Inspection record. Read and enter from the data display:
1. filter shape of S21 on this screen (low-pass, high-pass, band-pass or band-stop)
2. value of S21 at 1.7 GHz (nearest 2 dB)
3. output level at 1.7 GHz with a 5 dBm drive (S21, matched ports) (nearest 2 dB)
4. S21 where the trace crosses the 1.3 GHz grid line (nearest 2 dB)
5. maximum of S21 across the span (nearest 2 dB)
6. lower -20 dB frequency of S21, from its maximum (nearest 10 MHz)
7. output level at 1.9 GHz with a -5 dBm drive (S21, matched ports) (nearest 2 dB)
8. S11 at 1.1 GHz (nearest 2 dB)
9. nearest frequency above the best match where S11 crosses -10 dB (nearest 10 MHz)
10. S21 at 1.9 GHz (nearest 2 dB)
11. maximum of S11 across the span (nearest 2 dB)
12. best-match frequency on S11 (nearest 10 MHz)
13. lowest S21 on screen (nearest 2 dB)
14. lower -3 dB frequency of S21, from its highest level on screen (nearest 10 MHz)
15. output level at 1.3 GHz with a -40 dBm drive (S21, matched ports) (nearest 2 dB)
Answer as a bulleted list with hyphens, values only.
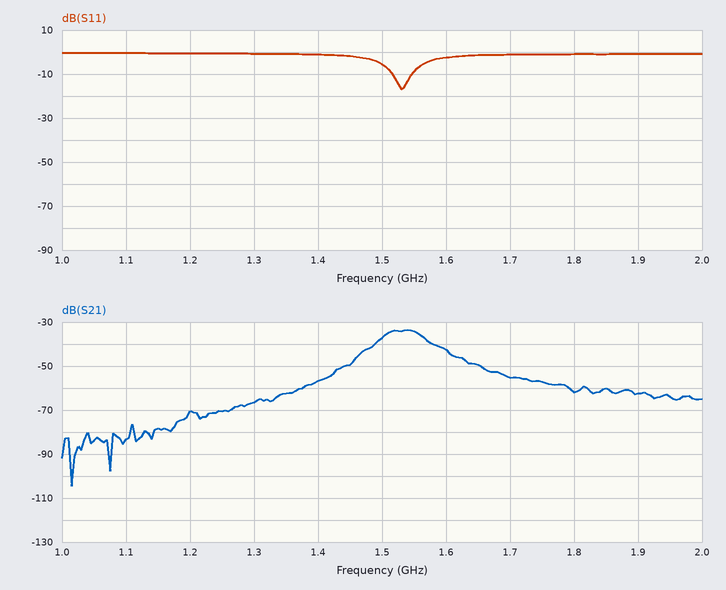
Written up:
- band-pass
- -56 dB
- -50 dBm
- -66 dB
- -34 dB
- 1.42 GHz
- -68 dBm
- 0 dB
- 1.55 GHz
- -62 dB
- 0 dB
- 1.53 GHz
- -104 dB
- 1.50 GHz
- -106 dBm
